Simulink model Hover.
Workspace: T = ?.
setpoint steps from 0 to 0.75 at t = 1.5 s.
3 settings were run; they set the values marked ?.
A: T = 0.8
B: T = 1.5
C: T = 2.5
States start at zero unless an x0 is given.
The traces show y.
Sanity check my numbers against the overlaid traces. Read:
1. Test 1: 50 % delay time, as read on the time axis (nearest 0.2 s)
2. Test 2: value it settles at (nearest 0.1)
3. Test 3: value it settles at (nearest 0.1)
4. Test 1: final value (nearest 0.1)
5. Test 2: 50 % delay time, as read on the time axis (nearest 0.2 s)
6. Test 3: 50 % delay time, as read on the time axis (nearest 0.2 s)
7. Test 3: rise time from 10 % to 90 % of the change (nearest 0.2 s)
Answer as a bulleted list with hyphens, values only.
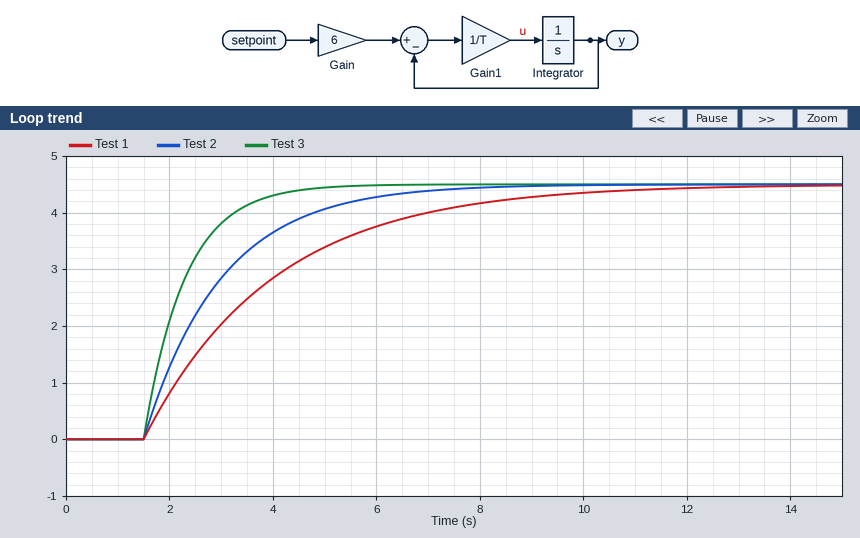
- 3.2 s
- 4.5
- 4.5
- 4.5
- 2.6 s
- 2.0 s
- 1.8 s
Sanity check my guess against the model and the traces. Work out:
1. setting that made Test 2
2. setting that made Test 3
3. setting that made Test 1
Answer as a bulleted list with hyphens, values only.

- B
- A
- C
